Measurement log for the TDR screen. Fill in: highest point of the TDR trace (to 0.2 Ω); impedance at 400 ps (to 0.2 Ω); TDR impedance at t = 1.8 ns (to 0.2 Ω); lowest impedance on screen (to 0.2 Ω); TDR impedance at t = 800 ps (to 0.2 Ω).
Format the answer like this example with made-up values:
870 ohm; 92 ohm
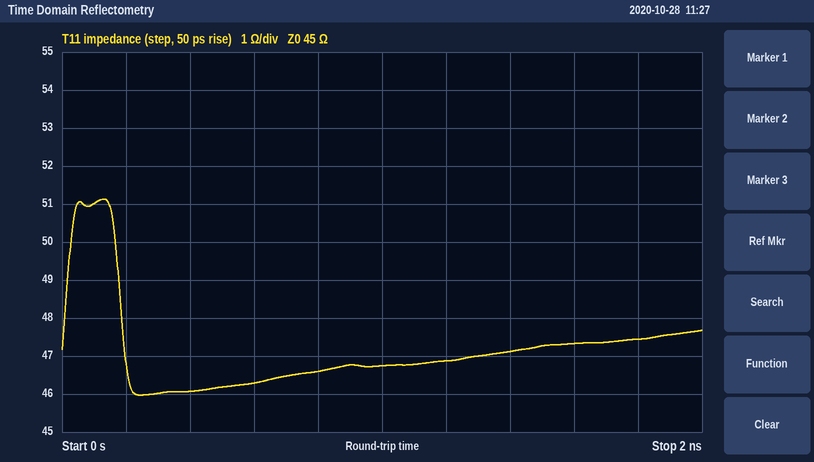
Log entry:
51.2 Ω; 46.0 Ω; 47.4 Ω; 46.0 Ω; 46.6 Ω
